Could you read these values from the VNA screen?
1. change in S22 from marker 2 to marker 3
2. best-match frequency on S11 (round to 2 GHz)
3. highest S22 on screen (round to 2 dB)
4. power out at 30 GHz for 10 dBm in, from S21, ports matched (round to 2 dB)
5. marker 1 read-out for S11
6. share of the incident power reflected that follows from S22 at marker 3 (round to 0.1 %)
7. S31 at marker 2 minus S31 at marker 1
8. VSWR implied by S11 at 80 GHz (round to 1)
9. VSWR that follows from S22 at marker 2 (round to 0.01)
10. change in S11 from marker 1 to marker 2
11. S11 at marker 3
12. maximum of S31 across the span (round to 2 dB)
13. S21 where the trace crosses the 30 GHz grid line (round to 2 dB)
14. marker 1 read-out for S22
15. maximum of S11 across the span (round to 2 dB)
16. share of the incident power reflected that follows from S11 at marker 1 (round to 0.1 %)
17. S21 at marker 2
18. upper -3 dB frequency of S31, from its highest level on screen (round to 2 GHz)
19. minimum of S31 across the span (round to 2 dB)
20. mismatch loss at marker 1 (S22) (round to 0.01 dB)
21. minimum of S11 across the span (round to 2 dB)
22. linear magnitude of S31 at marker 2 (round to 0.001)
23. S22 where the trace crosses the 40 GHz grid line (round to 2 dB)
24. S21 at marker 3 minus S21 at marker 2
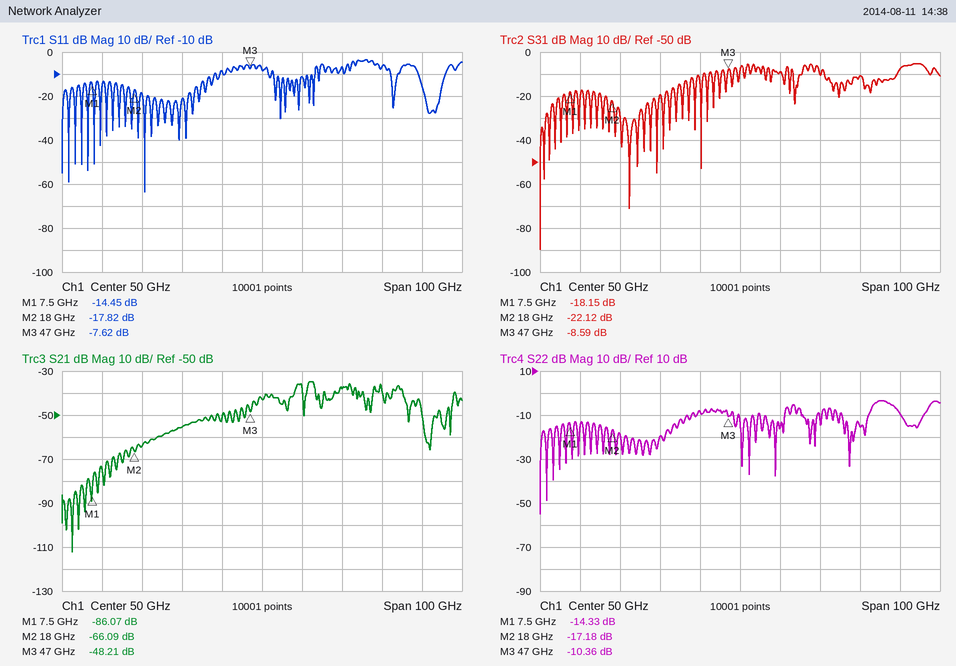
6.82 dB
20 GHz
-4 dB
-46 dBm
-14.45 dB
9.2 %
-3.97 dB
3
1.32
-3.37 dB
-7.62 dB
-6 dB
-56 dB
-14.33 dB
-4 dB
3.6 %
-66.09 dB
96 GHz
-90 dB
0.16 dB
-64 dB
0.078
-8 dB
17.88 dB
